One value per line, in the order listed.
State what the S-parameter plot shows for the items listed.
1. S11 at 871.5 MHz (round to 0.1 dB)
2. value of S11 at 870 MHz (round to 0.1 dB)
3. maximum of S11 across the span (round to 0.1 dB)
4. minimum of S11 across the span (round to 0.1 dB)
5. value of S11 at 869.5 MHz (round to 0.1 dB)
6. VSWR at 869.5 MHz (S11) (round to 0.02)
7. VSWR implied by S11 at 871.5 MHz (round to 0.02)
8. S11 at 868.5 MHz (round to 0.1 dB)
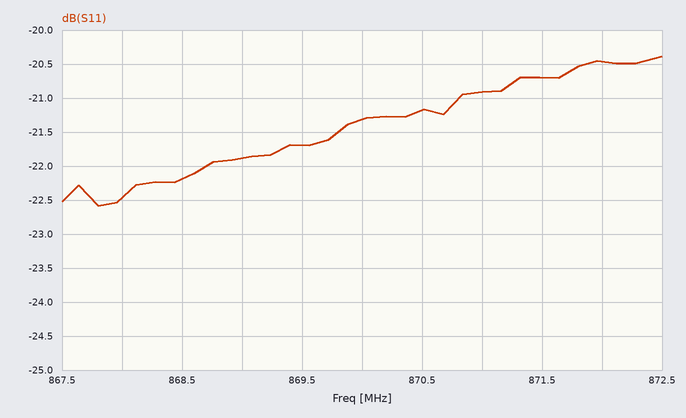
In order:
-20.7 dB
-21.3 dB
-20.4 dB
-22.6 dB
-21.7 dB
1.18
1.20
-22.2 dB
